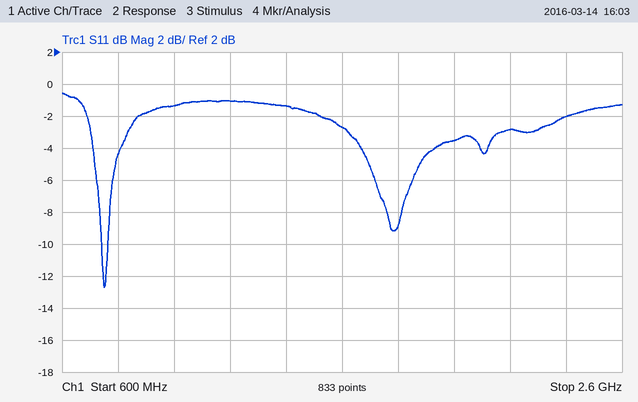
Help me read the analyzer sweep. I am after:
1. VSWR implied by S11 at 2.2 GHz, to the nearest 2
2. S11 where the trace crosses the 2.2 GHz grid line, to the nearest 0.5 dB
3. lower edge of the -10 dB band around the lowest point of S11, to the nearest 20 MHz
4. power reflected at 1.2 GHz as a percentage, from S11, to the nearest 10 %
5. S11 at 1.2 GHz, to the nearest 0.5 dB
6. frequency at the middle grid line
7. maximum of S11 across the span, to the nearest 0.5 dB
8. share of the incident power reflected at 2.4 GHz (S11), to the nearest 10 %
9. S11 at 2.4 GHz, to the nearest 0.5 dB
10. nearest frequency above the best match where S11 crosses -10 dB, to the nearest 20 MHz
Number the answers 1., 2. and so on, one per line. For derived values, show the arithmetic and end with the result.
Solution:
1. |Γ| = 10^(-3/20) = 0.7079; VSWR = (1 + 0.7079)/(1 − 0.7079) ≈ 6
2. -3.0 dB
3. 740 MHz
4. 10^(-1/10) ≈ 79.4 %, so 80 % to the nearest 10 %
5. -1.0 dB
6. 1.6 GHz
7. -0.5 dB
8. 10^(-2/10) ≈ 63.1 %, so 60 % to the nearest 10 %
9. -2.0 dB
10. 760 MHz
